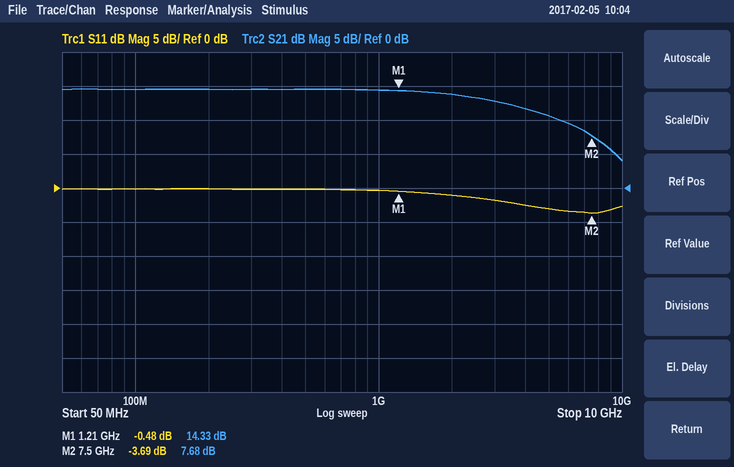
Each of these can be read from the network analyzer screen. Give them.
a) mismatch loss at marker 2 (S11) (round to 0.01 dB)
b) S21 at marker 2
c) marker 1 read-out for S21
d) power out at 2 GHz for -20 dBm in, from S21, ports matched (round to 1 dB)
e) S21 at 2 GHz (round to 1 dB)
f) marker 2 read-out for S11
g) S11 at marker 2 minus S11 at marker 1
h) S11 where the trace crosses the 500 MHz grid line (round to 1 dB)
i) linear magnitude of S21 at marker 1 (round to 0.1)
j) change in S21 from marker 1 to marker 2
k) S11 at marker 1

2.42 dB
7.68 dB
14.33 dB
-6 dBm
14 dB
-3.69 dB
-3.21 dB
0 dB
5.2
-6.65 dB
-0.48 dB
